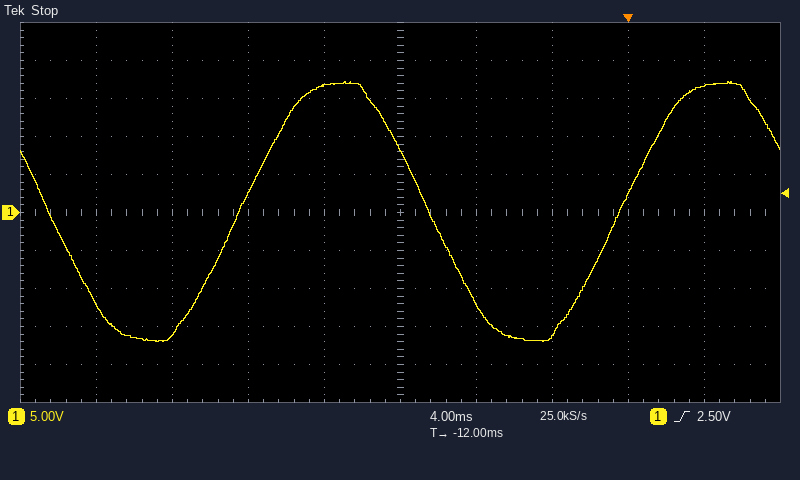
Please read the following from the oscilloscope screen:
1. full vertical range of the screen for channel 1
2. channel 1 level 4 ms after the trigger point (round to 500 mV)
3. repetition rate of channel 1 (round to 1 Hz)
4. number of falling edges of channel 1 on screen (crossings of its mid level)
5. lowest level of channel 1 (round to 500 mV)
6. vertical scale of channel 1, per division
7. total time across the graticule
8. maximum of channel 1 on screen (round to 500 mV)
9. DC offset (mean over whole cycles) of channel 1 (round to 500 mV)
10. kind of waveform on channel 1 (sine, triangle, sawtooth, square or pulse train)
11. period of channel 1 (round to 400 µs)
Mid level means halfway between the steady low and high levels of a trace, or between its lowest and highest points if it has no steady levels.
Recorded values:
50 V
16.5 V
50 Hz
2
-17.0 V
5 V
40 ms
17.0 V
0.0 V
sine
20.0 ms
